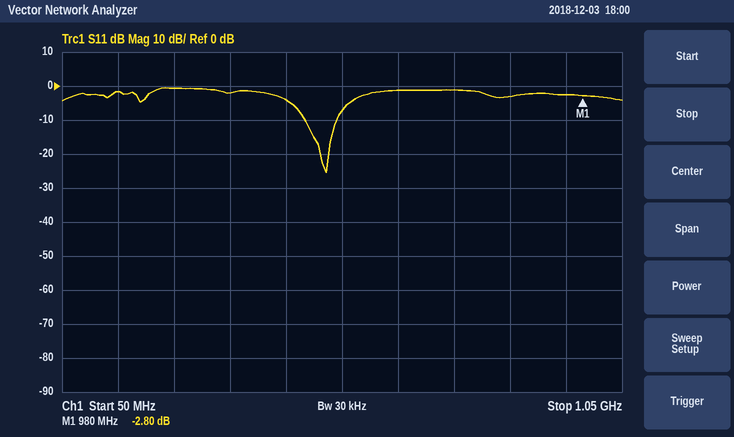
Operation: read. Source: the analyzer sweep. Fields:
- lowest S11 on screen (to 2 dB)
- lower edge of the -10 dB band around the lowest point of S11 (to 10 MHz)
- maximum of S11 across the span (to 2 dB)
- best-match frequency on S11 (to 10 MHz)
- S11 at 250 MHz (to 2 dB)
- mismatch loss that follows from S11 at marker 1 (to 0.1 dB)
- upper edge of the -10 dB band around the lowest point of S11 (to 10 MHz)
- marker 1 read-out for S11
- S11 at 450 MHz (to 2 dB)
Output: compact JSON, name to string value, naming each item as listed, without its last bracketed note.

{"lowest S11 on screen": "-26 dB", "lower edge of the -10 dB band around the lowest point of S11": "480 MHz", "maximum of S11 across the span": "0 dB", "best-match frequency on S11": "520 MHz", "S11 at 250 MHz": "0 dB", "mismatch loss that follows from S11 at marker 1": "3.2 dB", "upper edge of the -10 dB band around the lowest point of S11": "540 MHz", "marker 1 read-out for S11": "-2.80 dB", "S11 at 450 MHz": "-4 dB"}
